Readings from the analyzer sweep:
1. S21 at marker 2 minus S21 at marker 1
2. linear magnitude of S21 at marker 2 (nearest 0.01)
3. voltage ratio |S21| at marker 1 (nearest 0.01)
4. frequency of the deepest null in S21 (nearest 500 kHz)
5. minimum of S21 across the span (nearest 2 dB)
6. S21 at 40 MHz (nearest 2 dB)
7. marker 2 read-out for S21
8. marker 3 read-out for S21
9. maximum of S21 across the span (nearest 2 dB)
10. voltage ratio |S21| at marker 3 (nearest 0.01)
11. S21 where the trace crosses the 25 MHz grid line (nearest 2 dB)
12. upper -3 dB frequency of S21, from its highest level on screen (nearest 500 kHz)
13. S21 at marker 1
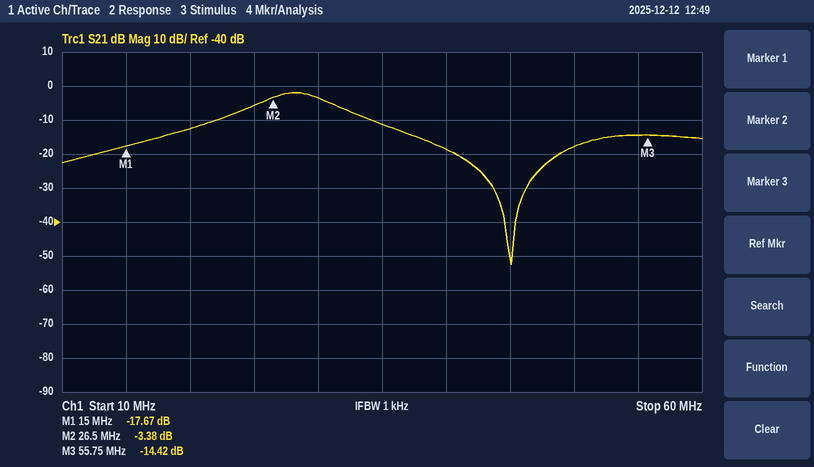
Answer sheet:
14.29 dB
0.68
0.13
45.0 MHz
-52 dB
-18 dB
-3.38 dB
-14.42 dB
-2 dB
0.19
-6 dB
31.0 MHz
-17.67 dB
